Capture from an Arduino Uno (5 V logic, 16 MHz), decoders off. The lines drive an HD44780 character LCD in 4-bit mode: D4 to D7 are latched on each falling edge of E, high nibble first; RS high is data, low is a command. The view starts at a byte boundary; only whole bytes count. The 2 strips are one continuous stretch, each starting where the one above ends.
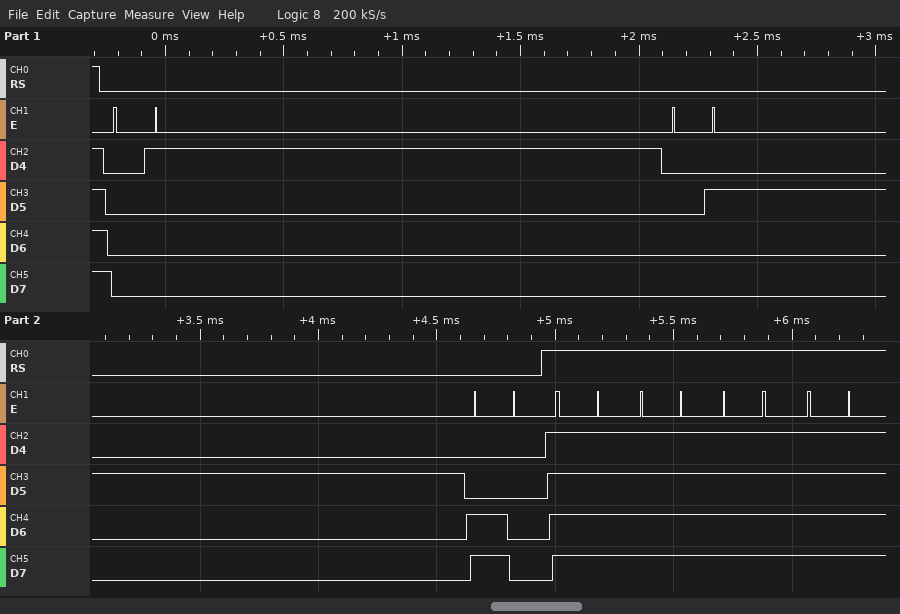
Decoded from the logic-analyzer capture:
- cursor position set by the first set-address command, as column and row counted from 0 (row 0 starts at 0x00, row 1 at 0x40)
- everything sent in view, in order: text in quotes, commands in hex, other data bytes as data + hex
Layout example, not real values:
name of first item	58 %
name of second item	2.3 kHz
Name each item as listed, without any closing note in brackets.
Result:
cursor position set by the first set-address command, as column and row counted from 0	column 0, row 1
everything sent in view, in order: text in quotes, commands in hex, other data bytes as data + hex	0x01 0x02 0xC0 data FF FF FF FF
